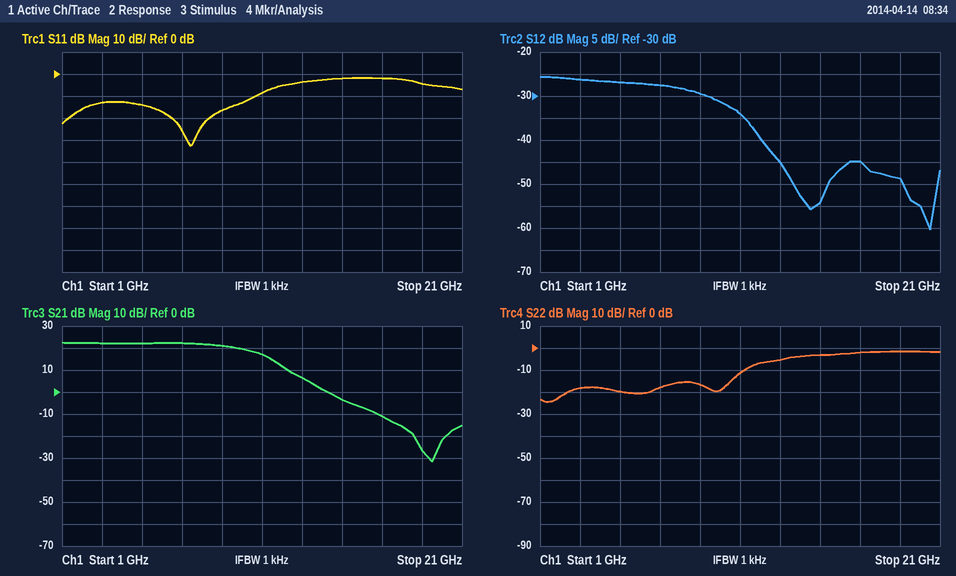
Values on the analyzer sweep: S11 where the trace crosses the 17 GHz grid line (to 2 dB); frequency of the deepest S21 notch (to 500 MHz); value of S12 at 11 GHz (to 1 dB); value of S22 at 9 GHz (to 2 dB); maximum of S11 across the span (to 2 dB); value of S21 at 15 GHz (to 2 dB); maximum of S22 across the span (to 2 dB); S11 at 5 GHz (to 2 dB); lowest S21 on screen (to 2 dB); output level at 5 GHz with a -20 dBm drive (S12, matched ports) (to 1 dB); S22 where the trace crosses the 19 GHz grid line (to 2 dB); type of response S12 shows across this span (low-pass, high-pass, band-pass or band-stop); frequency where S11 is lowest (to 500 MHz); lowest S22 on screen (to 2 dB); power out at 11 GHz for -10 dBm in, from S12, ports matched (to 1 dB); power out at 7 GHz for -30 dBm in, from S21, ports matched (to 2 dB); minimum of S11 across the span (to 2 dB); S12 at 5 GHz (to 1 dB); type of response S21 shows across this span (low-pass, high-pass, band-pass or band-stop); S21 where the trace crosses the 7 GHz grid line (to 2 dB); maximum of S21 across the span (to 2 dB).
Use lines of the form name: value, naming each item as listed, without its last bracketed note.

S11 where the trace crosses the 17 GHz grid line: -2 dB
frequency of the deepest S21 notch: 19.5 GHz
value of S12 at 11 GHz: -34 dB
value of S22 at 9 GHz: -16 dB
maximum of S11 across the span: -2 dB
value of S21 at 15 GHz: -4 dB
maximum of S22 across the span: -2 dB
S11 at 5 GHz: -14 dB
lowest S21 on screen: -32 dB
output level at 5 GHz with a -20 dBm drive (S12, matched ports): -47 dBm
S22 where the trace crosses the 19 GHz grid line: -2 dB
type of response S12 shows across this span: low-pass
frequency where S11 is lowest: 7.5 GHz
lowest S22 on screen: -24 dB
power out at 11 GHz for -10 dBm in, from S12, ports matched: -44 dBm
power out at 7 GHz for -30 dBm in, from S21, ports matched: -8 dBm
minimum of S11 across the span: -32 dB
S12 at 5 GHz: -27 dB
type of response S21 shows across this span: low-pass
S21 where the trace crosses the 7 GHz grid line: 22 dB
maximum of S21 across the span: 22 dB
